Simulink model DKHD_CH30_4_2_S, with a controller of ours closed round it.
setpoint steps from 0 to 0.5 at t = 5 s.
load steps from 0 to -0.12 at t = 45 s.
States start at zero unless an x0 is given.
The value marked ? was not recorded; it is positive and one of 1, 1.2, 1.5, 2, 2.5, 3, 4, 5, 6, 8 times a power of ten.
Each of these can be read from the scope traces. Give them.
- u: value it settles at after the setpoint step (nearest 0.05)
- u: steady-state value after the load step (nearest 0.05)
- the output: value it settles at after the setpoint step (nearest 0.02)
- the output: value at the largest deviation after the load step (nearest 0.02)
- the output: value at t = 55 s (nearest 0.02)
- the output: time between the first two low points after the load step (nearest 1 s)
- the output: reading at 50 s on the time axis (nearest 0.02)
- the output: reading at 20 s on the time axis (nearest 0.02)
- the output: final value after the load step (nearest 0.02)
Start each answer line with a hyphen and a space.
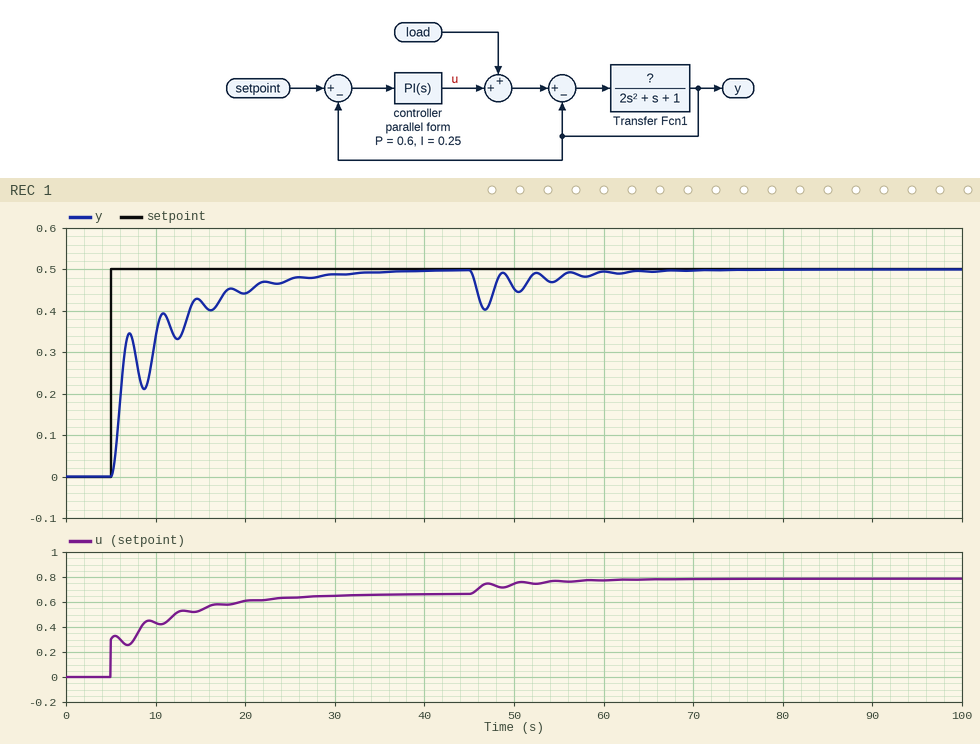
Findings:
- 0.65
- 0.80
- 0.50
- 0.40
- 0.48
- 4 s
- 0.46
- 0.44
- 0.50
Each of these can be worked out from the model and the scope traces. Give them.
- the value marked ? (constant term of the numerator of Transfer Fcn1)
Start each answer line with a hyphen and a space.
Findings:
- 3
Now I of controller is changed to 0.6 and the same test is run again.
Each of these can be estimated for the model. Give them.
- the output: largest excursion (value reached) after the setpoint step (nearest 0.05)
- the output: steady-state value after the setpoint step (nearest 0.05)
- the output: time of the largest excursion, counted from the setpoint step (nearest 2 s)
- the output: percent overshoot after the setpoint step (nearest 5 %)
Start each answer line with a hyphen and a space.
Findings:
- 0.55
- 0.50
- 10 s
- 10 %
